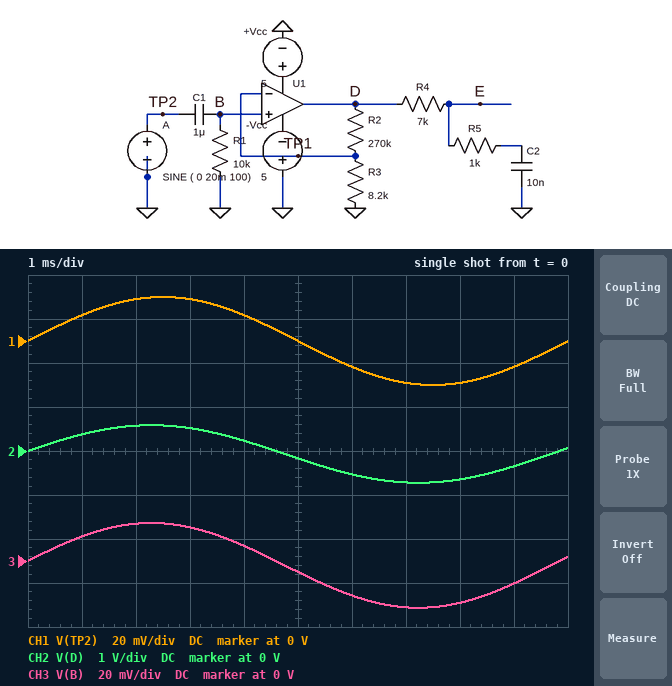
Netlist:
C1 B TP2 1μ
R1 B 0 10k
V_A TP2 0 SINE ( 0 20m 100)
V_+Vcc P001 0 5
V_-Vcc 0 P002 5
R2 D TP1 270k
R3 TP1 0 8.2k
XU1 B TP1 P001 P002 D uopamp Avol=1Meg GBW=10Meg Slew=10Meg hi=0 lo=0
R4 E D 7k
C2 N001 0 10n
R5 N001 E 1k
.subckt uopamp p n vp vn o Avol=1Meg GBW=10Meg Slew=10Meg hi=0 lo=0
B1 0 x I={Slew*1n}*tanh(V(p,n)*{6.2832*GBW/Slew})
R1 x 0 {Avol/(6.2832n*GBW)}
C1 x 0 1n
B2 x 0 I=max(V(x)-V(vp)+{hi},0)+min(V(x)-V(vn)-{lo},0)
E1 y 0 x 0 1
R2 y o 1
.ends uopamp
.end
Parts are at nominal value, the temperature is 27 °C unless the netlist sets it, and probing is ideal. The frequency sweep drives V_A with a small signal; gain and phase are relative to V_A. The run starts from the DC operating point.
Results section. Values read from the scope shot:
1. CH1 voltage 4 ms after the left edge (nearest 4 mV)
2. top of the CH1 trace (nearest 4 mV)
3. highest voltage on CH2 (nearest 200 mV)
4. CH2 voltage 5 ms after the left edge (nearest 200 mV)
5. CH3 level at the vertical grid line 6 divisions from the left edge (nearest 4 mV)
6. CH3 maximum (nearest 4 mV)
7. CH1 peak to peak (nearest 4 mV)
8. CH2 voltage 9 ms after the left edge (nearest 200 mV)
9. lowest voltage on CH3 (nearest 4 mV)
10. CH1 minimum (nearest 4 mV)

12 mV
20 mV
600 mV
-200 mV
-16 mV
16 mV
40 mV
-400 mV
-20 mV
-20 mV
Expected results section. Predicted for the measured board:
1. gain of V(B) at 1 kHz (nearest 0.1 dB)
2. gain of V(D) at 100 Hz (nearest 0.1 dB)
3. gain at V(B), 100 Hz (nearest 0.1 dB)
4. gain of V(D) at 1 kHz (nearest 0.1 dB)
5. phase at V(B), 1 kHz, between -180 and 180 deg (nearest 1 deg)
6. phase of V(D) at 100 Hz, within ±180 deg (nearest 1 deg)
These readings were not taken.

0 dB
30.5 dB
-0.1 dB
30.6 dB
1 deg
9 deg
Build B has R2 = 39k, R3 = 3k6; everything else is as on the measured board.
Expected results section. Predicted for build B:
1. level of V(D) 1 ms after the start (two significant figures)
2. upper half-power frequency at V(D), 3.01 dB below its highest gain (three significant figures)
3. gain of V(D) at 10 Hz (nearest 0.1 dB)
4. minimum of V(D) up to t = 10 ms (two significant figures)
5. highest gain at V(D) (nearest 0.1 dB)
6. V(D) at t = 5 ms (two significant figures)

130 mV
845 kHz
16.0 dB
-250 mV
21.5 dB
-59 mV
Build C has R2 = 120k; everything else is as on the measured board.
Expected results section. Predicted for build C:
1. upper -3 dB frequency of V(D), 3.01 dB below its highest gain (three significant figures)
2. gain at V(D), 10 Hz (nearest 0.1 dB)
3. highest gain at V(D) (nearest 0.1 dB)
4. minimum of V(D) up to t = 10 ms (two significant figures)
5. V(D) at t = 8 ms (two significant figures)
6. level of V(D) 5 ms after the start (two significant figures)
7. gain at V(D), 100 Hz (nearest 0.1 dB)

640 kHz
18.4 dB
23.9 dB
-330 mV
-300 mV
-78 mV
23.8 dB
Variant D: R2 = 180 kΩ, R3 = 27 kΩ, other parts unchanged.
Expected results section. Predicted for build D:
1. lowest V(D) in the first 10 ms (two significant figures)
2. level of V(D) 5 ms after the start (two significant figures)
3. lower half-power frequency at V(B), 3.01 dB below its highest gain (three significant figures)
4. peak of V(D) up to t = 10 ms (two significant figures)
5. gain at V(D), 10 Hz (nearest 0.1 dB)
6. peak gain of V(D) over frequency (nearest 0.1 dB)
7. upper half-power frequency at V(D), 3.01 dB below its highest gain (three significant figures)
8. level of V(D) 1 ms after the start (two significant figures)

-160 mV
-38 mV
15.9 Hz
130 mV
12.2 dB
17.7 dB
1.30 MHz
86 mV
